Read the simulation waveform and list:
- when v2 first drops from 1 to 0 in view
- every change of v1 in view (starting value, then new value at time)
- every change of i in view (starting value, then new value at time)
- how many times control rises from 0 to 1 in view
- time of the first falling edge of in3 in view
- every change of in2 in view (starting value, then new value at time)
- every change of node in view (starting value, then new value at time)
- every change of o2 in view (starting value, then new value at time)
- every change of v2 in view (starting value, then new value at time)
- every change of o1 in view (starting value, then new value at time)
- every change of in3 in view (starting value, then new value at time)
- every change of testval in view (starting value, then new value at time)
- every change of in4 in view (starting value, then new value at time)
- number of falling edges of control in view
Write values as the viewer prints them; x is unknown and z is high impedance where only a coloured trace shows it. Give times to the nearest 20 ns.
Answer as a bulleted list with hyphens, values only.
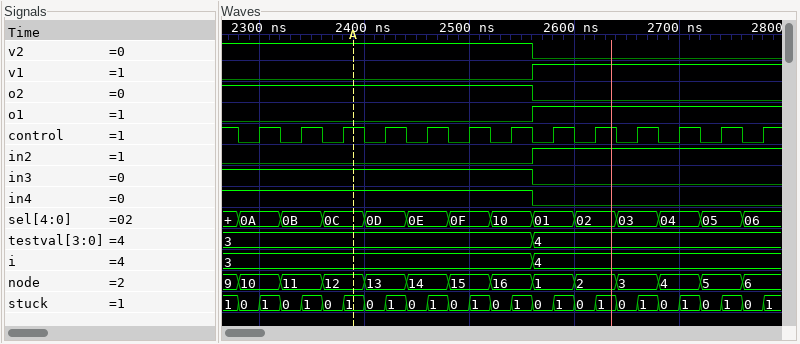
- 2560 ns
- 0, 1 at 2560 ns
- 3, 4 at 2560 ns
- 13
- 2560 ns
- 0, 1 at 2560 ns
- 9, 10 at 2280 ns, 11 at 2320 ns, 12 at 2360 ns, 13 at 2400 ns, 14 at 2440 ns, 15 at 2480 ns, 16 at 2520 ns, 1 at 2560 ns, 2 at 2600 ns, 3 at 2640 ns, 4 at 2680 ns, 5 at 2720 ns, 6 at 2760 ns
- 1, 0 at 2560 ns
- 1, 0 at 2560 ns
- 0, 1 at 2560 ns
- 1, 0 at 2560 ns
- 3, 4 at 2560 ns
- 1, 0 at 2560 ns
- 13
